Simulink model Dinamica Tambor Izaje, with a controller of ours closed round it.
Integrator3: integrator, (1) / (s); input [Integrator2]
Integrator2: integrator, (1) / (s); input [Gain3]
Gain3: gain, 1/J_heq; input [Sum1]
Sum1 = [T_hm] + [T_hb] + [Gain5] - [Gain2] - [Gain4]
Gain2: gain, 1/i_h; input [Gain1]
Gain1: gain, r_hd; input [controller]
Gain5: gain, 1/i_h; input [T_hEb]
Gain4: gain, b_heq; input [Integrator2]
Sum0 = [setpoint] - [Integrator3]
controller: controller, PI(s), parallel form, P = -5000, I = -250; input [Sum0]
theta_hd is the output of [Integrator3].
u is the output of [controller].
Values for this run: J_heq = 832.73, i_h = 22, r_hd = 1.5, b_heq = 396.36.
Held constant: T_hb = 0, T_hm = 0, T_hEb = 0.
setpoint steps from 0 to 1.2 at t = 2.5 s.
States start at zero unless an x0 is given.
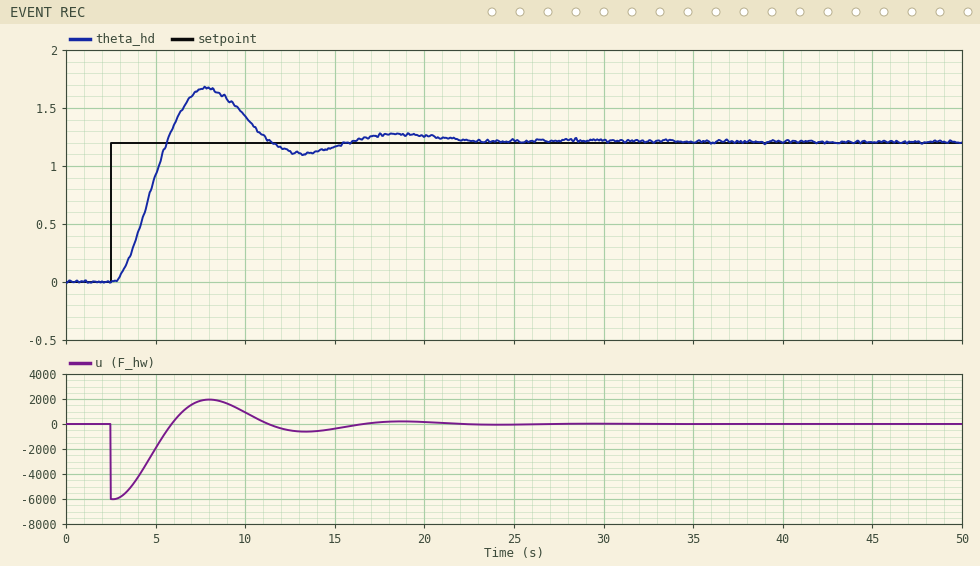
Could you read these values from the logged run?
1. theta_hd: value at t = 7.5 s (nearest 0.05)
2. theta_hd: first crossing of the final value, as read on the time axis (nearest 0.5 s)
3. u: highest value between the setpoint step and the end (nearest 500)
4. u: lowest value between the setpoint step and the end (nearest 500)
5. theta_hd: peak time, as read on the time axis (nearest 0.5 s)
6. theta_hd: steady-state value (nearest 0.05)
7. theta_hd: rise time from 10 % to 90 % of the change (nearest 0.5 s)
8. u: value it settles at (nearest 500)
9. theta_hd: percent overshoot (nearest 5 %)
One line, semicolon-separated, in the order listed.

1.65; 5.5 s; 2000; -6000; 8.0 s; 1.20; 2.0 s; 0; 40 %
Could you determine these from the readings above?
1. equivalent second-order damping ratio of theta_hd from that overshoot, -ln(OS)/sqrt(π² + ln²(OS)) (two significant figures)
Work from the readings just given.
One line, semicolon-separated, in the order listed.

0.28
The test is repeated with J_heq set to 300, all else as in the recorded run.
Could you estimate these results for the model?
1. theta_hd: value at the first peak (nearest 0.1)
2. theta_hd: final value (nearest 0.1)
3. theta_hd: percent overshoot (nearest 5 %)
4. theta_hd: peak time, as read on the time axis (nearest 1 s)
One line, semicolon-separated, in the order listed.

1.4; 1.2; 15 %; 6 s
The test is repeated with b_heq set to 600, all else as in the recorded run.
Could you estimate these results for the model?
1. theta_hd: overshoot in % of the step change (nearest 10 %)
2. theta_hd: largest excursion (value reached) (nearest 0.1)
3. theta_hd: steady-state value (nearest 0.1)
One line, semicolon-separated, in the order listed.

20 %; 1.5; 1.2
